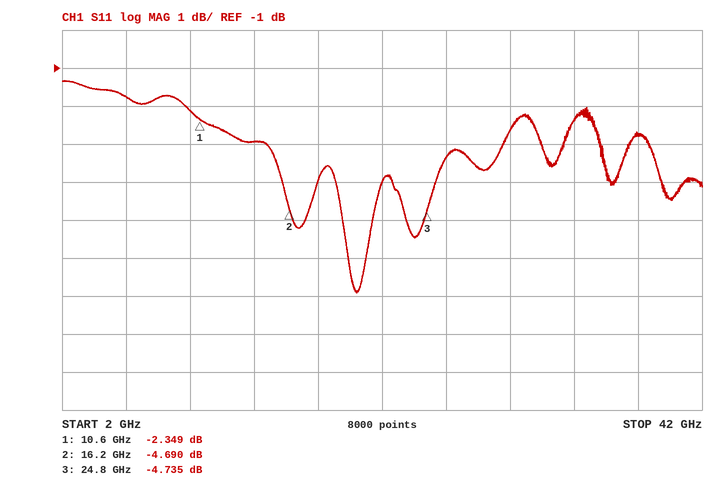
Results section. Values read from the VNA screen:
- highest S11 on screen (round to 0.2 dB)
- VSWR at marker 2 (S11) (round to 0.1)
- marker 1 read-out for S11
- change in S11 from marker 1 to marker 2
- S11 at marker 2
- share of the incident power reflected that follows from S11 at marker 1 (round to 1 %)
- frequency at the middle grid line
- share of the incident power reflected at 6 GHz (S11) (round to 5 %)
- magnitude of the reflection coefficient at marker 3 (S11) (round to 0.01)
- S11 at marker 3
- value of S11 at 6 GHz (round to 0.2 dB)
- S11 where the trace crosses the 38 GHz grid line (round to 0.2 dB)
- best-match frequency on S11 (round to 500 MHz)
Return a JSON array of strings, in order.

["-1.4 dB", "3.8", "-2.349 dB", "-2.341 dB", "-4.690 dB", "58 %", "22 GHz", "65 %", "0.58", "-4.735 dB", "-1.8 dB", "-2.8 dB", "20.5 GHz"]
